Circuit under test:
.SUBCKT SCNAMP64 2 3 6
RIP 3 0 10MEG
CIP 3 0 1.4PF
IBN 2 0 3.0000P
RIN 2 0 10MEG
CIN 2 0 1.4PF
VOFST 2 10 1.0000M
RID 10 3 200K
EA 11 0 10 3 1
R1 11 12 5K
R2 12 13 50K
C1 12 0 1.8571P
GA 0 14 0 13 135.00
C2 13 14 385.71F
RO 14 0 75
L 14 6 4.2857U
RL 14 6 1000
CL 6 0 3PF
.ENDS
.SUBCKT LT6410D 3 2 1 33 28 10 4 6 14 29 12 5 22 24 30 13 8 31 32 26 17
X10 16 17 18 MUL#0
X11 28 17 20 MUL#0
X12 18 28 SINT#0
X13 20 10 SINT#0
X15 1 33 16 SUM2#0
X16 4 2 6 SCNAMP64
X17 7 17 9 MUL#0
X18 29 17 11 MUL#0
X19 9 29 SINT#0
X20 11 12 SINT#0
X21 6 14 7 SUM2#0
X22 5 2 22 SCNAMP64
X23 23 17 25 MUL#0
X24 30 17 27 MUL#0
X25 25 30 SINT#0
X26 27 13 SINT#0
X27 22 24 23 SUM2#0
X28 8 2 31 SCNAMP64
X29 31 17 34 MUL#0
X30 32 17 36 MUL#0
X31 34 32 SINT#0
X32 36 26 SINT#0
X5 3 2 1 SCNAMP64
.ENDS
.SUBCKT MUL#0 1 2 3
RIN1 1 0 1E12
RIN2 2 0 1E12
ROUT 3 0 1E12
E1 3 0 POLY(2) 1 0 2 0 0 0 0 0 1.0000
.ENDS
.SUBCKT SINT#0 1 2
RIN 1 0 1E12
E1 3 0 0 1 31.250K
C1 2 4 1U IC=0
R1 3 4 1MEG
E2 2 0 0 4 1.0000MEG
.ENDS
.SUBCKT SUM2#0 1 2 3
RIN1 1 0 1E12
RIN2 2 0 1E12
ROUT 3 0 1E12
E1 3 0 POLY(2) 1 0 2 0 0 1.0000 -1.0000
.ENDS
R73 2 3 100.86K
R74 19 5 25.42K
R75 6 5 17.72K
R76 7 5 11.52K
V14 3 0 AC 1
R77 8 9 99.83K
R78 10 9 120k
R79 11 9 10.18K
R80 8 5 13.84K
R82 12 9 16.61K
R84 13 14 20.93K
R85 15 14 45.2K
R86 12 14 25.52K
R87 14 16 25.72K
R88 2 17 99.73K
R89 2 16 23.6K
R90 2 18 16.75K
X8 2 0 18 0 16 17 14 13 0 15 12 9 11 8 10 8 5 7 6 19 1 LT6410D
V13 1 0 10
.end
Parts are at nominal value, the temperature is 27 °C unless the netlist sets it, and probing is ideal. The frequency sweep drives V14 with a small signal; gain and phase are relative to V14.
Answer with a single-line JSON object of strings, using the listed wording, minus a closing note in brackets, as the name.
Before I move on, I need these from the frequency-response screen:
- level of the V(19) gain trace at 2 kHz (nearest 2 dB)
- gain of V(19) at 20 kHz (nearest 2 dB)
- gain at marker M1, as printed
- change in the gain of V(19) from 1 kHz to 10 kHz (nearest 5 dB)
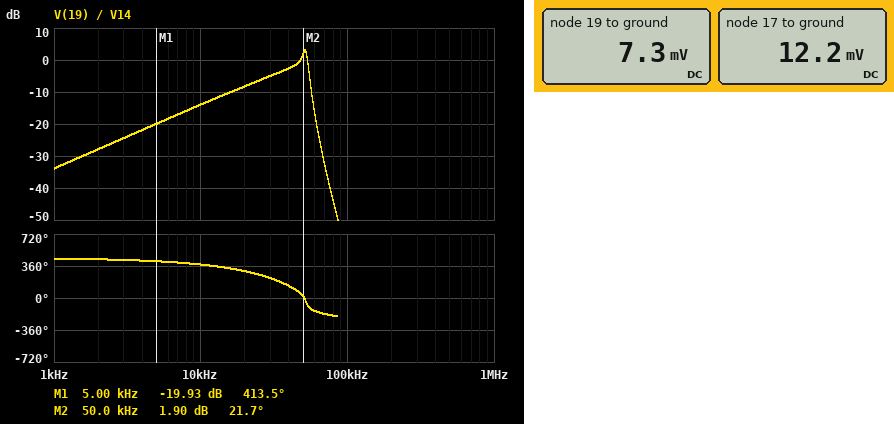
{"level of the V(19) gain trace at 2 kHz": "-28 dB", "gain of V(19) at 20 kHz": "-8 dB", "gain at marker M1, as printed": "-19.93 dB", "change in the gain of V(19) from 1 kHz to 10 kHz": "20 dB"}
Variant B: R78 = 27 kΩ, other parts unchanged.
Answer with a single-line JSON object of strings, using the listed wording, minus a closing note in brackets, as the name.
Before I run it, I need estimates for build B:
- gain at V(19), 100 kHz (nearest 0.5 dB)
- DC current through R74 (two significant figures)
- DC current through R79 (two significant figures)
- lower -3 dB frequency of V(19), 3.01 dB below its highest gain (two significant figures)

{"gain at V(19), 100 kHz": "-61.0 dB", "DC current through R74": "230 nA", "DC current through R79": "120 nA", "lower -3 dB frequency of V(19), 3.01 dB below its highest gain": "23 kHz"}
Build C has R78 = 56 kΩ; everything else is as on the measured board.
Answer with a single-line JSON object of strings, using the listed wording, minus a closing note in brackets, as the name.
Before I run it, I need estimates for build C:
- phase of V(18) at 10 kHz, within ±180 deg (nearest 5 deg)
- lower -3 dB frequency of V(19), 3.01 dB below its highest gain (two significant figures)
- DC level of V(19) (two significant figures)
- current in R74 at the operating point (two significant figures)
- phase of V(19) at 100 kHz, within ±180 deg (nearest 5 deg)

{"phase of V(18) at 10 kHz, within ±180 deg": "-50 deg", "lower -3 dB frequency of V(19), 3.01 dB below its highest gain": "29 kHz", "DC level of V(19)": "7.2 mV", "current in R74 at the operating point": "240 nA", "phase of V(19) at 100 kHz, within ±180 deg": "145 deg"}
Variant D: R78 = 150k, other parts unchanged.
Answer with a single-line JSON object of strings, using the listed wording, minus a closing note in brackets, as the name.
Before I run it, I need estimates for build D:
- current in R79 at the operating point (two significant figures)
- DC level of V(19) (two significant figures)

{"current in R79 at the operating point": "150 nA", "DC level of V(19)": "7.4 mV"}
